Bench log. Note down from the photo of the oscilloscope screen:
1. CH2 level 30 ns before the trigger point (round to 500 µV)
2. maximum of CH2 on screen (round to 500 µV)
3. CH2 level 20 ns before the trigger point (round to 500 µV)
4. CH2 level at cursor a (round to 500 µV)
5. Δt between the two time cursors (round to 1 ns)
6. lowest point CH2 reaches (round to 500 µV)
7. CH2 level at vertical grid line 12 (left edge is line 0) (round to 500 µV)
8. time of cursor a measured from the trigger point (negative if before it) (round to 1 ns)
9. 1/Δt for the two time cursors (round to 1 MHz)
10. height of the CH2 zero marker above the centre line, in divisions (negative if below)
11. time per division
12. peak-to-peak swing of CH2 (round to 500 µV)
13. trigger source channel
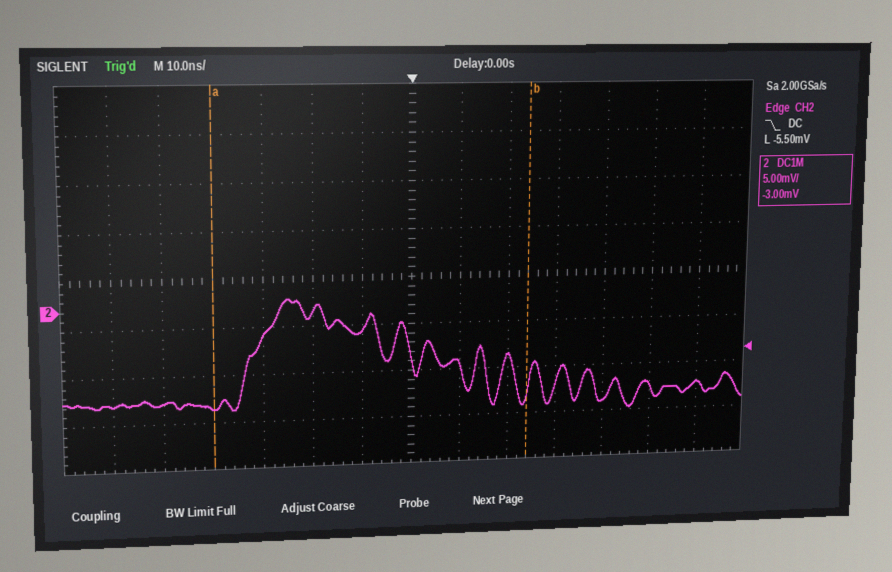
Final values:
-3.0 mV
1.0 mV
-500 µV
-10.5 mV
64 ns
-11.5 mV
-9.5 mV
-40 ns
16 MHz
-0.6 div
10 ns
12.5 mV
CH2
